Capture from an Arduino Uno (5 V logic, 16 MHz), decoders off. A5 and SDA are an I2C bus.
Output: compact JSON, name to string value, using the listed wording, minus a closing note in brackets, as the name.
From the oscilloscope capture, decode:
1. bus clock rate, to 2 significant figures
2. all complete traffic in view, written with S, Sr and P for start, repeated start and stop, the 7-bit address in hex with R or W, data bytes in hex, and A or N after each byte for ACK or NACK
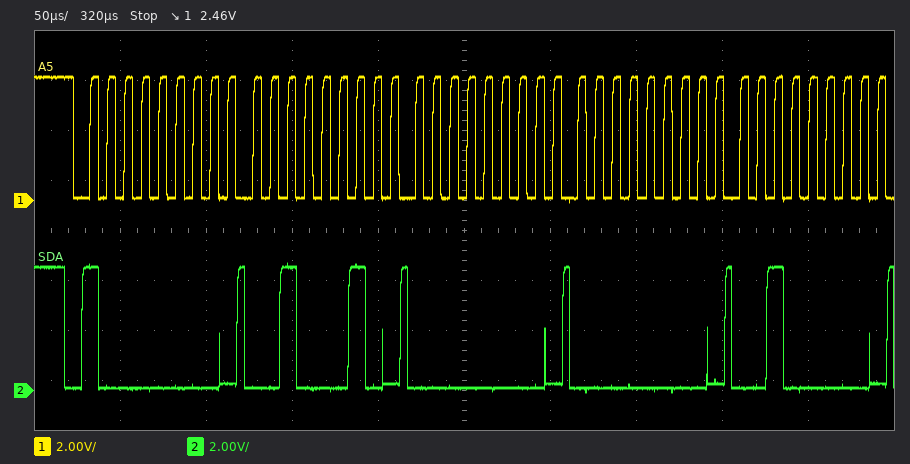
{"bus clock rate, to 2 significant figures": "100 kHz", "all complete traffic in view, written with S, Sr and P for start, repeated start and stop, the 7-bit address in hex with R or W, data bytes in hex, and A or N after each byte for ACK or NACK": "S 40W A 22 A 00 A 00 A 20 A"}
